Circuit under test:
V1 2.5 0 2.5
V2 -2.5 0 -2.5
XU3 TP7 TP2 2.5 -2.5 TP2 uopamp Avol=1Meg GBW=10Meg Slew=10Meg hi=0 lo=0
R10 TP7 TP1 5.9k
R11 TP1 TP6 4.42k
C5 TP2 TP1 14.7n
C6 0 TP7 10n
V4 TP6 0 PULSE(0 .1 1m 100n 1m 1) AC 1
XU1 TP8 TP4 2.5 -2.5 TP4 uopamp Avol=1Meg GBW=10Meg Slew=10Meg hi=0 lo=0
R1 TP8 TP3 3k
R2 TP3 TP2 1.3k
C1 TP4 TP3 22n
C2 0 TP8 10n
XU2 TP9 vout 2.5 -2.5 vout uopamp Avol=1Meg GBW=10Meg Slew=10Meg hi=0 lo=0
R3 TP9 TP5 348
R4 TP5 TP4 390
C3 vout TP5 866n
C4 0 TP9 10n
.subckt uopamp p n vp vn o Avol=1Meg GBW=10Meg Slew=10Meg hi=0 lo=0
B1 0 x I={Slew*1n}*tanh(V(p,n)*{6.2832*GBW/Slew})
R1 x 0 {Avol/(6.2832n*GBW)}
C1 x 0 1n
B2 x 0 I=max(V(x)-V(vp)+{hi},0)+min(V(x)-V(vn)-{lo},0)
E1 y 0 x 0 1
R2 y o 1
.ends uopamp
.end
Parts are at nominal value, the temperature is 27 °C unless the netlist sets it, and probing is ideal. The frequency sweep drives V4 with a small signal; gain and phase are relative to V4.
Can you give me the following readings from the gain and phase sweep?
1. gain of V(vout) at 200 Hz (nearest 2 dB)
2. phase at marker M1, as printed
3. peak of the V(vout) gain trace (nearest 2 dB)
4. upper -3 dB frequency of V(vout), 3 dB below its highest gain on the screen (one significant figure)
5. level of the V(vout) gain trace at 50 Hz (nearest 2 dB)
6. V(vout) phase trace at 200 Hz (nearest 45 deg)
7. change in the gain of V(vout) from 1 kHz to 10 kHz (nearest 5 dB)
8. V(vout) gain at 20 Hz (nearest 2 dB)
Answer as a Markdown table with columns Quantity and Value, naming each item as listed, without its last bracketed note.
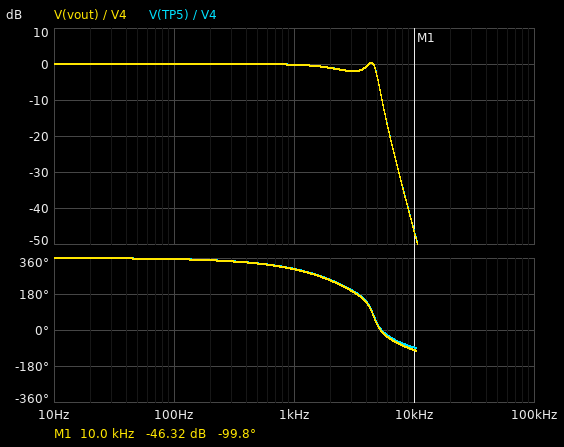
| Quantity | Value |
|---|---|
| gain of V(vout) at 200 Hz | 0 dB |
| phase at marker M1, as printed | -99.8 deg |
| peak of the V(vout) gain trace | 0 dB |
| upper -3 dB frequency of V(vout), 3 dB below its highest gain on the screen | 5 kHz |
| level of the V(vout) gain trace at 50 Hz | 0 dB |
| V(vout) phase trace at 200 Hz | 360 deg |
| change in the gain of V(vout) from 1 kHz to 10 kHz | -45 dB |
| V(vout) gain at 20 Hz | 0 dB |
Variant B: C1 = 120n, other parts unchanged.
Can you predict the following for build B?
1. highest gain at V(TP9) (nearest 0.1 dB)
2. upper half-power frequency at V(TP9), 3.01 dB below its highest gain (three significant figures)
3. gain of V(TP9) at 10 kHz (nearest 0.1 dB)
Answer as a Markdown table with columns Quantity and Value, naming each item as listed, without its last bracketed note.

| Quantity | Value |
|---|---|
| highest gain at V(TP9) | 3.5 dB |
| upper half-power frequency at V(TP9), 3.01 dB below its highest gain | 2.69 kHz |
| gain of V(TP9) at 10 kHz | -60.1 dB |
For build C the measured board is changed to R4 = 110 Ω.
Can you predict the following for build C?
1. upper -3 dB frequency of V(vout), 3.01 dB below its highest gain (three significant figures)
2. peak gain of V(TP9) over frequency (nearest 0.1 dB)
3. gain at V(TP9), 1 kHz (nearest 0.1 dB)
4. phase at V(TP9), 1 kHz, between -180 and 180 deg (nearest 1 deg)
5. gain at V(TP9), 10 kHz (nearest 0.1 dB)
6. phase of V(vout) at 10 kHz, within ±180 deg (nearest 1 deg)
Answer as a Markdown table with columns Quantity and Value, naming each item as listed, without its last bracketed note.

| Quantity | Value |
|---|---|
| upper -3 dB frequency of V(vout), 3.01 dB below its highest gain | 2.24 kHz |
| peak gain of V(TP9) over frequency | 0 dB |
| gain at V(TP9), 1 kHz | -0.5 dB |
| phase at V(TP9), 1 kHz, between -180 and 180 deg | -55 deg |
| gain at V(TP9), 10 kHz | -27.6 dB |
| phase of V(vout) at 10 kHz, within ±180 deg | -65 deg |
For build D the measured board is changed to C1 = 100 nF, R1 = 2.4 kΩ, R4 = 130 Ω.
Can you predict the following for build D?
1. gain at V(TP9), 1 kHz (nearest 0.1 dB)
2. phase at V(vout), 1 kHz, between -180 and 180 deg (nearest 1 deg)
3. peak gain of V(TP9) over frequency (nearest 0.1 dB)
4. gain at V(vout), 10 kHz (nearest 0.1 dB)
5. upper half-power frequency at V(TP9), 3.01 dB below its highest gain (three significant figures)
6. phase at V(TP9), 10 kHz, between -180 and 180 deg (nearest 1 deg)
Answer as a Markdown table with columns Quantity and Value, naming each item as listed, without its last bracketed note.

| Quantity | Value |
|---|---|
| gain at V(TP9), 1 kHz | 0.4 dB |
| phase at V(vout), 1 kHz, between -180 and 180 deg | -54 deg |
| peak gain of V(TP9) over frequency | 1.2 dB |
| gain at V(vout), 10 kHz | -41.1 dB |
| upper half-power frequency at V(TP9), 3.01 dB below its highest gain | 3.03 kHz |
| phase at V(TP9), 10 kHz, between -180 and 180 deg | -115 deg |
